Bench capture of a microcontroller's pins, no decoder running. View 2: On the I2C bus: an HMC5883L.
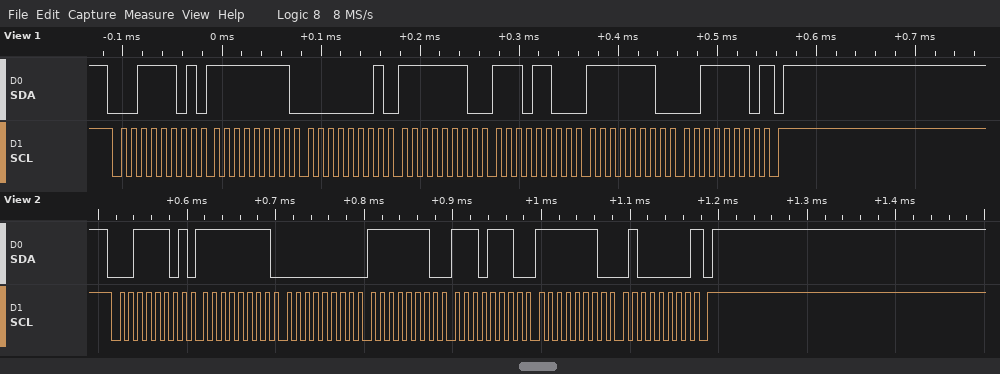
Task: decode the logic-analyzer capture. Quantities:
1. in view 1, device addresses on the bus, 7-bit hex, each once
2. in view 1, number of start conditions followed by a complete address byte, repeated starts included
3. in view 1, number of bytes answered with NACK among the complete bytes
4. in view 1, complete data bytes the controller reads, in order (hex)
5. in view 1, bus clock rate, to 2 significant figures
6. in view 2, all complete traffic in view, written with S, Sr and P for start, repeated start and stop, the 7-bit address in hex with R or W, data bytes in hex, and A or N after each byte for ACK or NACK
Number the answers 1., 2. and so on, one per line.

1. 0x1E
2. 1
3. 1
4. FF 01 FE EC FE 3E
5. 100 kHz
6. S 1ER A FF A 00 A FE A EE A FE A 40 N P
